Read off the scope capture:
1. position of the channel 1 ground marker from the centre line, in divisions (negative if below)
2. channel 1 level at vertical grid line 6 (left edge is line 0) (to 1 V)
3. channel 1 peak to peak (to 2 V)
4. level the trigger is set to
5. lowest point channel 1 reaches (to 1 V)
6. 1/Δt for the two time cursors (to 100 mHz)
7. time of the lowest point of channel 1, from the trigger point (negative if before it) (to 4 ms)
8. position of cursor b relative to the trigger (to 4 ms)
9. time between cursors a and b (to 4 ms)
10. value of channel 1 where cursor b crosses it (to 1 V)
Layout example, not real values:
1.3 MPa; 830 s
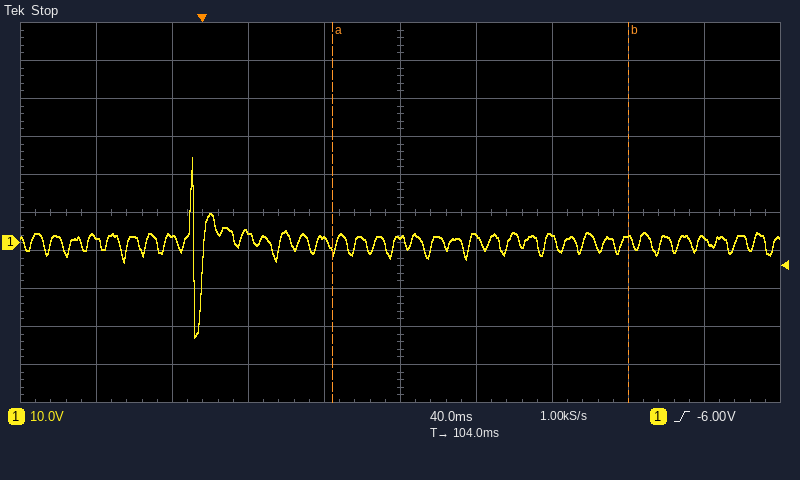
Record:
-0.8 div; 2 V; 48 V; -6.00 V; -25 V; 6.4 Hz; -4 ms; +224 ms; 156 ms; 1 V
